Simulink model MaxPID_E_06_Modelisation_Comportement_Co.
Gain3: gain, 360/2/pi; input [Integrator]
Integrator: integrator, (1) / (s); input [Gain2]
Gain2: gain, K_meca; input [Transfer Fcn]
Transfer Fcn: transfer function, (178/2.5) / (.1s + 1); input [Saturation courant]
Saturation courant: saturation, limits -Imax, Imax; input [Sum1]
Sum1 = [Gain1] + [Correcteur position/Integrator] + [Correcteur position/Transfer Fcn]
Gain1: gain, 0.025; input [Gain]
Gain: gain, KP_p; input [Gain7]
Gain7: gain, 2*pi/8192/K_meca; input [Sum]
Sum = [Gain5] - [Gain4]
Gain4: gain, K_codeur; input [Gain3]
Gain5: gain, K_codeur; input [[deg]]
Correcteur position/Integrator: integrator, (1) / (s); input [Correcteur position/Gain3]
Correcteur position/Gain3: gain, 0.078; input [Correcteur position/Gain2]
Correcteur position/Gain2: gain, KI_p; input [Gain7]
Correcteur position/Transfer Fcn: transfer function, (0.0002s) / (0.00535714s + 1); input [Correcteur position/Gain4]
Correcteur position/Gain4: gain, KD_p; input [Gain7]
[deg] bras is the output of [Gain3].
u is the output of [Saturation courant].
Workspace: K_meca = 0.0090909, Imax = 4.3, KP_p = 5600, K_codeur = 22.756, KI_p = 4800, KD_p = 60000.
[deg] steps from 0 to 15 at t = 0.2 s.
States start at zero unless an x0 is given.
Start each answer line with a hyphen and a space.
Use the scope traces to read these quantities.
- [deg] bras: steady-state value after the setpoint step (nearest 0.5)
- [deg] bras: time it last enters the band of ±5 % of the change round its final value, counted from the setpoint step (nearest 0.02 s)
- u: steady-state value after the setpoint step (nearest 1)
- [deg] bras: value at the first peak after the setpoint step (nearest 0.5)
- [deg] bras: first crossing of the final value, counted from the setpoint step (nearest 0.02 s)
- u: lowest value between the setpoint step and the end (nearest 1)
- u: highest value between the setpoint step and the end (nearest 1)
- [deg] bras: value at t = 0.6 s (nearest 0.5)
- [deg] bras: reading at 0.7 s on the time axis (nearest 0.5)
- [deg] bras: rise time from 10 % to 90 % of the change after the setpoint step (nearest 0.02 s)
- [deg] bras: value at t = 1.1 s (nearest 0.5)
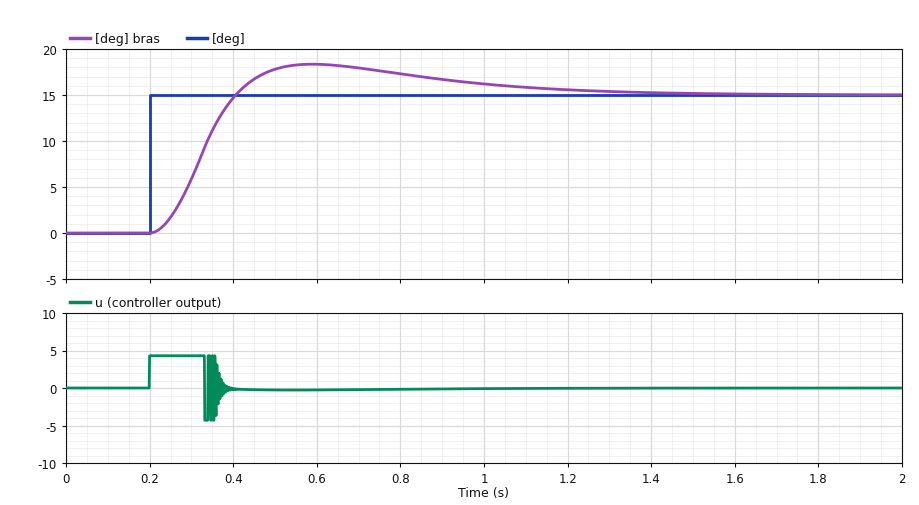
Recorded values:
- 15.0
- 0.92 s
- 0
- 18.5
- 0.20 s
- -4
- 4
- 18.5
- 18.0
- 0.14 s
- 16.0
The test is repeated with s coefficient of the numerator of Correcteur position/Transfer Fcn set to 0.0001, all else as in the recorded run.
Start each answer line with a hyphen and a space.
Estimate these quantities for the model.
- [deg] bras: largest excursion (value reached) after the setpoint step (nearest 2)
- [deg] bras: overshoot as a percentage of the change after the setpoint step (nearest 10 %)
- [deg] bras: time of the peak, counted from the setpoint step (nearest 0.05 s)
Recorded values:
- 18
- 20 %
- 0.30 s
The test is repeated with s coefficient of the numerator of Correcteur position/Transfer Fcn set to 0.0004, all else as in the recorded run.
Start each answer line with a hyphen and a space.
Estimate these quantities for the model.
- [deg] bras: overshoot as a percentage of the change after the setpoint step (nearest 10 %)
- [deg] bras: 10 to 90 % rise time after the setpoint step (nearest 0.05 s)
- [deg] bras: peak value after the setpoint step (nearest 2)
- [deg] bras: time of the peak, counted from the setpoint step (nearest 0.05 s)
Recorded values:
- 20 %
- 0.20 s
- 18
- 0.55 s
